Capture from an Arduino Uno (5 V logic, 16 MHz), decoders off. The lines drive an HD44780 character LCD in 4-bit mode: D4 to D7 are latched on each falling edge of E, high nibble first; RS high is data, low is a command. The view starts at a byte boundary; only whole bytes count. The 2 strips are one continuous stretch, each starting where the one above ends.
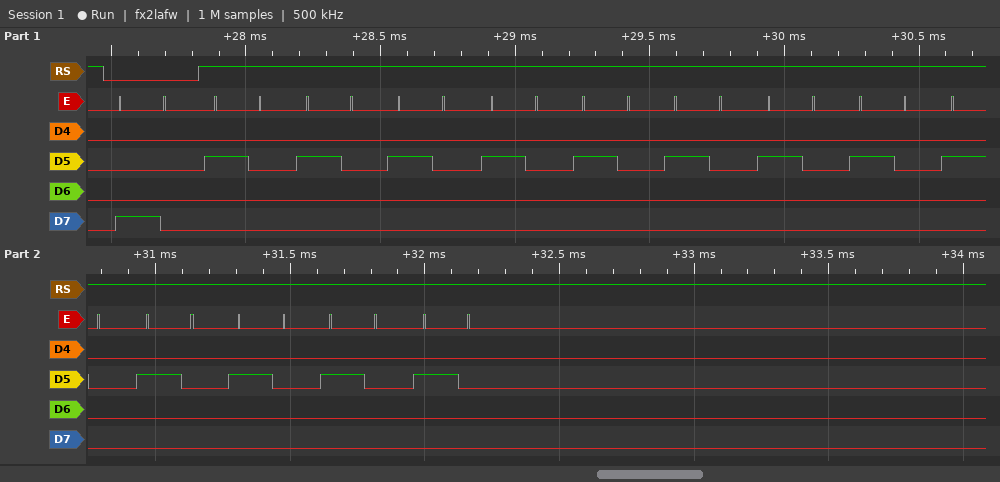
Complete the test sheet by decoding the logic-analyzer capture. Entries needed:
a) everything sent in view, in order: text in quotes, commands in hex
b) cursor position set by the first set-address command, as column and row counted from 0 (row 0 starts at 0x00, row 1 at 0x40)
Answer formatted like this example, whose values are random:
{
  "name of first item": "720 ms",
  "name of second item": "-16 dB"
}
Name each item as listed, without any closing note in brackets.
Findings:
{
  "everything sent in view, in order: text in quotes, commands in hex": "0x80 \"             \"",
  "cursor position set by the first set-address command, as column and row counted from 0": "column 0, row 0"
}
